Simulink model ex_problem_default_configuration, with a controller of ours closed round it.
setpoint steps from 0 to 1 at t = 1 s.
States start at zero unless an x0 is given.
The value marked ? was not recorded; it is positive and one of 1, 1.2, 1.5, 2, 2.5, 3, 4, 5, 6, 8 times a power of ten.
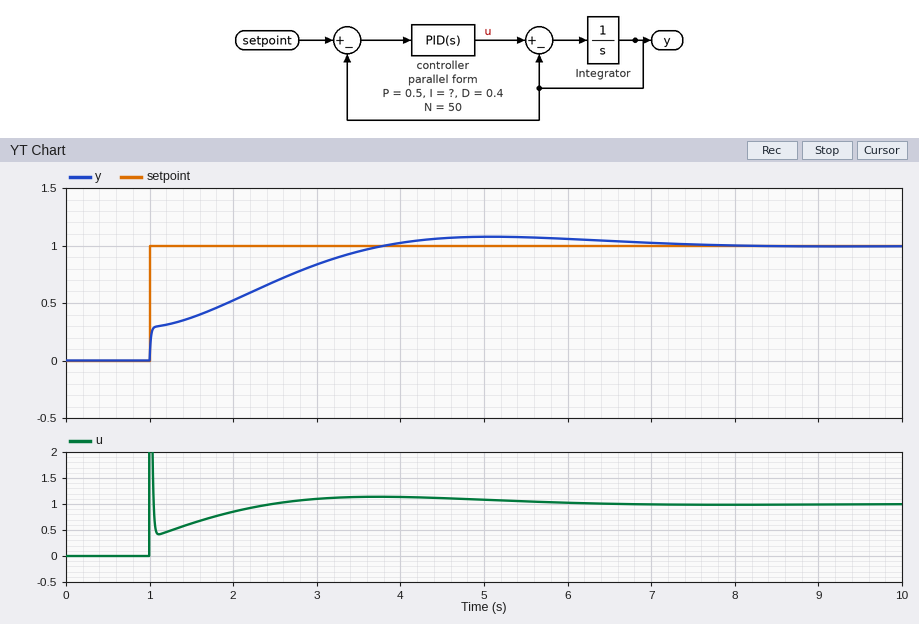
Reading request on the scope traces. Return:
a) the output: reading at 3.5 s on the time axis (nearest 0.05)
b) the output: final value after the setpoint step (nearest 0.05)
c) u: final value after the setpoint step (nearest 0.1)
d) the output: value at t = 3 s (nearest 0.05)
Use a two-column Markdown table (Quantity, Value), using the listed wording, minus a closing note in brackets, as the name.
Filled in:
| Quantity | Value |
|---|---|
| the output: reading at 3.5 s on the time axis | 0.95 |
| the output: final value after the setpoint step | 1.00 |
| u: final value after the setpoint step | 1.0 |
| the output: value at t = 3 s | 0.85 |
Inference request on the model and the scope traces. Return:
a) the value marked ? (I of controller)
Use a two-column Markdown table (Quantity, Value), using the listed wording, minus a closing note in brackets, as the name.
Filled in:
| Quantity | Value |
|---|---|
| the value marked ? | 1.2 |
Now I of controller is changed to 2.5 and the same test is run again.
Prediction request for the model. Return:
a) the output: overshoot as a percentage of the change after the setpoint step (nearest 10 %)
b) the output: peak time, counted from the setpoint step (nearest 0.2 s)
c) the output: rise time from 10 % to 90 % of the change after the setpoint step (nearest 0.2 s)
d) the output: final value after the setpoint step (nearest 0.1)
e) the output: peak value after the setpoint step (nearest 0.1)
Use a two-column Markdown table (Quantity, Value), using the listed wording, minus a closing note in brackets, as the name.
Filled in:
| Quantity | Value |
|---|---|
| the output: overshoot as a percentage of the change after the setpoint step | 20 % |
| the output: peak time, counted from the setpoint step | 2.6 s |
| the output: rise time from 10 % to 90 % of the change after the setpoint step | 1.4 s |
| the output: final value after the setpoint step | 1.0 |
| the output: peak value after the setpoint step | 1.2 |
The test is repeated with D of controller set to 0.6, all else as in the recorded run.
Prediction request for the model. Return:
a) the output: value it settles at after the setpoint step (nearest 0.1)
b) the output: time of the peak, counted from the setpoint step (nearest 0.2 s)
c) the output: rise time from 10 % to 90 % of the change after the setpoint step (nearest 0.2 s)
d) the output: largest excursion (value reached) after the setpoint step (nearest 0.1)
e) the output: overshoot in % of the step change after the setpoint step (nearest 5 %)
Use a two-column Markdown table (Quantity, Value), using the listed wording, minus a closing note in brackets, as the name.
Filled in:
| Quantity | Value |
|---|---|
| the output: value it settles at after the setpoint step | 1.0 |
| the output: time of the peak, counted from the setpoint step | 4.4 s |
| the output: rise time from 10 % to 90 % of the change after the setpoint step | 2.4 s |
| the output: largest excursion (value reached) after the setpoint step | 1.1 |
| the output: overshoot in % of the step change after the setpoint step | 10 % |
